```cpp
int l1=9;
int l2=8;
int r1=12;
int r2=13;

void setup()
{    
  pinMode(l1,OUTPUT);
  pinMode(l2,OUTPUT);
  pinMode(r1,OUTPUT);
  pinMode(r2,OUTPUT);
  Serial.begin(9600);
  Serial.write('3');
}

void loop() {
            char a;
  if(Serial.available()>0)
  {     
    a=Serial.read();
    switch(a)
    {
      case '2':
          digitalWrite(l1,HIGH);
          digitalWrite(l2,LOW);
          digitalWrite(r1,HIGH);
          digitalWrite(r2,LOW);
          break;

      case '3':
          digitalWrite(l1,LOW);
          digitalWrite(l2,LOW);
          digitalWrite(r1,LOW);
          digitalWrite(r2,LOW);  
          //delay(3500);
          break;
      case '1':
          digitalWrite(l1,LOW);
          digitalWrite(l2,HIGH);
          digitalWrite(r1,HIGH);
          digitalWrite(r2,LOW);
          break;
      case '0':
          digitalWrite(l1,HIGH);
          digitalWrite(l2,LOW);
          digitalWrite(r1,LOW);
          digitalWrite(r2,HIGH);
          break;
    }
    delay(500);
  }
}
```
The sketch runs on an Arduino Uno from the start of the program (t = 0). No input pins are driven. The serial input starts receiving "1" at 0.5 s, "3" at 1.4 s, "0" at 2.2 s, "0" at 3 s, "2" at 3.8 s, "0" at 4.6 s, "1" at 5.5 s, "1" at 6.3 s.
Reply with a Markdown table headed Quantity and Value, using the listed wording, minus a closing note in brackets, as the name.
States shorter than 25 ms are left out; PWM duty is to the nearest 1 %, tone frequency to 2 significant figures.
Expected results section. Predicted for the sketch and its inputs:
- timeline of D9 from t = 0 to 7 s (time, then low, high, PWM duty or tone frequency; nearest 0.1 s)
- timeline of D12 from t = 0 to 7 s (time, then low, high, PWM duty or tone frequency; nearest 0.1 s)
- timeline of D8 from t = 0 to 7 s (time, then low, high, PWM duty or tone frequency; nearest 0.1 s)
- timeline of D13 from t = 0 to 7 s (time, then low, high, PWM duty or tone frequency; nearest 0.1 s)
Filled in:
| Quantity | Value |
|---|---|
| timeline of D9 from t = 0 to 7 s | 0 s low; 2.2 s high; 5.5 s low |
| timeline of D12 from t = 0 to 7 s | 0 s low; 0.5 s high; 1.4 s low; 3.8 s high; 4.6 s low; 5.5 s high |
| timeline of D8 from t = 0 to 7 s | 0 s low; 0.5 s high; 1.4 s low; 5.5 s high |
| timeline of D13 from t = 0 to 7 s | 0 s low; 2.2 s high; 3.8 s low; 4.6 s high; 5.5 s low |
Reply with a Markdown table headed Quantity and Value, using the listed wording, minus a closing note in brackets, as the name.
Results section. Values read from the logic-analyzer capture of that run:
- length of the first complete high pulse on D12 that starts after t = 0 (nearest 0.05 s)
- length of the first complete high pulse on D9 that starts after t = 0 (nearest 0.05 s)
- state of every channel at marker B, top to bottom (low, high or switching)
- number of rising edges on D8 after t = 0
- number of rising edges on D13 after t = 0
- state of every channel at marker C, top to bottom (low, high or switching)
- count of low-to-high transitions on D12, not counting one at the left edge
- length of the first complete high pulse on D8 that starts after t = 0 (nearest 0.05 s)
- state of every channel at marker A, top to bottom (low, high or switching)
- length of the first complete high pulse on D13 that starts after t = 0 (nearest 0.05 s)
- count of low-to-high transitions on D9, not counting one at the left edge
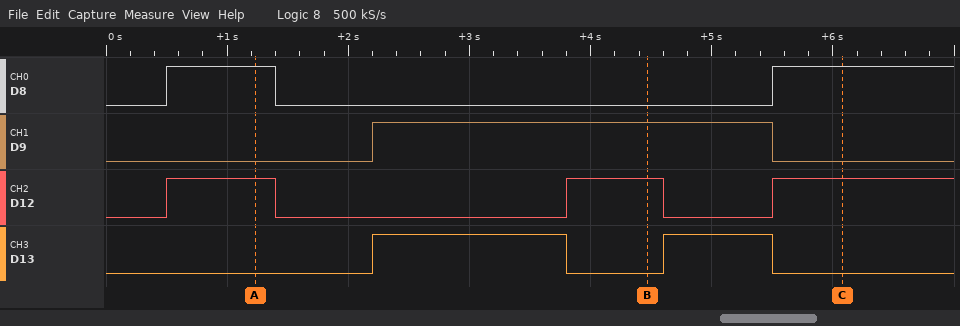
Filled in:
| Quantity | Value |
|---|---|
| length of the first complete high pulse on D12 that starts after t = 0 | 0.90 s |
| length of the first complete high pulse on D9 that starts after t = 0 | 3.30 s |
| state of every channel at marker B, top to bottom | D8 low, D9 high, D12 high, D13 low |
| number of rising edges on D8 after t = 0 | 2 |
| number of rising edges on D13 after t = 0 | 2 |
| state of every channel at marker C, top to bottom | D8 high, D9 low, D12 high, D13 low |
| count of low-to-high transitions on D12, not counting one at the left edge | 3 |
| length of the first complete high pulse on D8 that starts after t = 0 | 0.90 s |
| state of every channel at marker A, top to bottom | D8 high, D9 low, D12 high, D13 low |
| length of the first complete high pulse on D13 that starts after t = 0 | 1.60 s |
| count of low-to-high transitions on D9, not counting one at the left edge | 1 |
